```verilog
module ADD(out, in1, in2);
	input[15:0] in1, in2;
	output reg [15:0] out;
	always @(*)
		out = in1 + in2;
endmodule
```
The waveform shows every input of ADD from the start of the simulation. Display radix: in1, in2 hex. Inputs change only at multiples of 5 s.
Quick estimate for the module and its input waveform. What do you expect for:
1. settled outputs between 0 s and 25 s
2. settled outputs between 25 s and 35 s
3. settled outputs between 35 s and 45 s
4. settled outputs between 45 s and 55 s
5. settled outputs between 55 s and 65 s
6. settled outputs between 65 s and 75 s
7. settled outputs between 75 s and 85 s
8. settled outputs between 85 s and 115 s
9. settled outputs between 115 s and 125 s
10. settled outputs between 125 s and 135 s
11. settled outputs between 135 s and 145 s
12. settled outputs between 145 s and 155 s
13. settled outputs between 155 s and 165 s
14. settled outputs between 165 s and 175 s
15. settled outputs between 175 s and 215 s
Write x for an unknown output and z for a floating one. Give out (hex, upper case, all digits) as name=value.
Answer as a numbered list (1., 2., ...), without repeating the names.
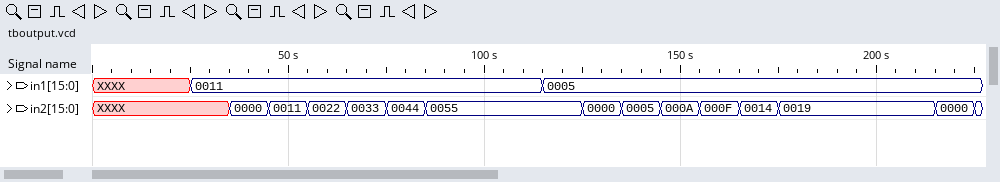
1. out=x
2. out=x
3. out=0011
4. out=0022
5. out=0033
6. out=0044
7. out=0055
8. out=0066
9. out=005A
10. out=0005
11. out=000A
12. out=000F
13. out=0014
14. out=0019
15. out=001E
